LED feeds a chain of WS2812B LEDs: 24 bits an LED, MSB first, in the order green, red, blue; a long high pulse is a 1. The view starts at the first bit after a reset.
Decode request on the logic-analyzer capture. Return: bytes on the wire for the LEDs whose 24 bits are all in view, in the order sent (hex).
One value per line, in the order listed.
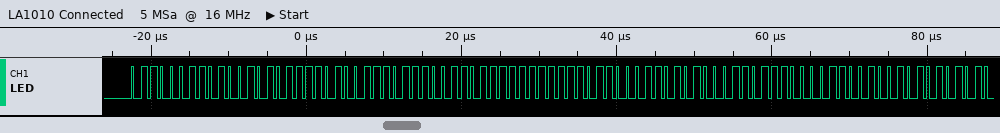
63 4A F4 EE 6F FE C6 A3 70
